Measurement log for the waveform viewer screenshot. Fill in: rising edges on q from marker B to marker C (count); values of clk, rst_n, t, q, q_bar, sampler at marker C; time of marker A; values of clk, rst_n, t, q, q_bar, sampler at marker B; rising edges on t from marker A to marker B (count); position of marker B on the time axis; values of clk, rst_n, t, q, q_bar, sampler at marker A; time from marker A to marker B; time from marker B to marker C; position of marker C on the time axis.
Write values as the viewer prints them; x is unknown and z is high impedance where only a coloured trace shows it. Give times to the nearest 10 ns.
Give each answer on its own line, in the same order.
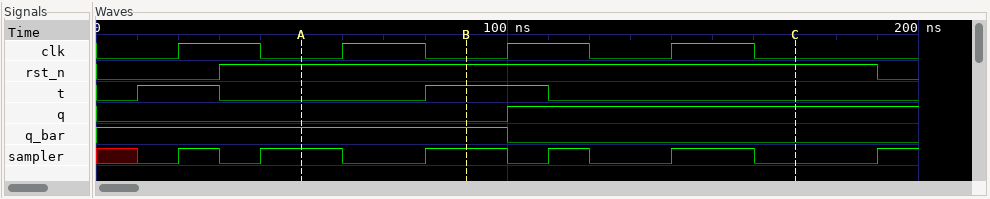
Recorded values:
1
clk=0, rst_n=1, t=0, q=1, q_bar=0, sampler=0
50 ns
clk=0, rst_n=1, t=1, q=0, q_bar=1, sampler=1
1
90 ns
clk=0, rst_n=1, t=0, q=0, q_bar=1, sampler=1
40 ns
80 ns
170 ns
